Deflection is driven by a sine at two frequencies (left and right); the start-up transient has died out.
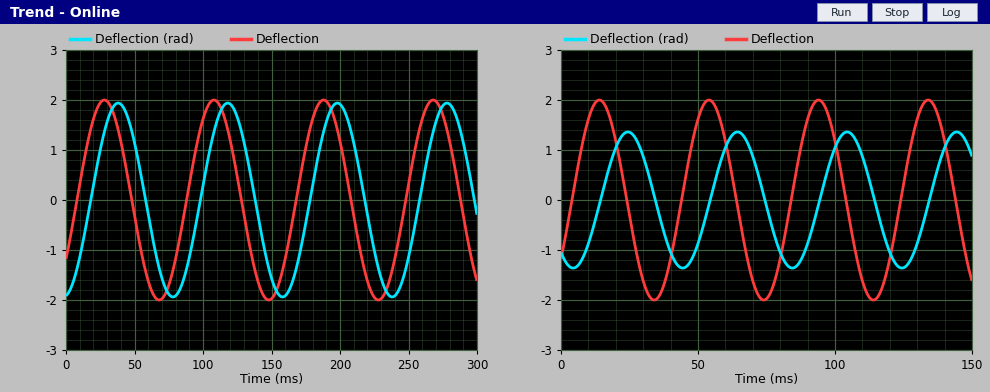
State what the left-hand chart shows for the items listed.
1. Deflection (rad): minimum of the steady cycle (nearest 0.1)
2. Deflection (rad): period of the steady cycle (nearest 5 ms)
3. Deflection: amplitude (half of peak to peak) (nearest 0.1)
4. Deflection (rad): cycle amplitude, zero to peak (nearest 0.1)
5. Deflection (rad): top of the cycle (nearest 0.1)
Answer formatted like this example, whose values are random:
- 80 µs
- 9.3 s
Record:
- -1.9
- 80 ms
- 2.0
- 1.9
- 1.9
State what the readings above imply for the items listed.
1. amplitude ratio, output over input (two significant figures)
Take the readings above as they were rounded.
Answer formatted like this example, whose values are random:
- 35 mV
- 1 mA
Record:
- 0.95
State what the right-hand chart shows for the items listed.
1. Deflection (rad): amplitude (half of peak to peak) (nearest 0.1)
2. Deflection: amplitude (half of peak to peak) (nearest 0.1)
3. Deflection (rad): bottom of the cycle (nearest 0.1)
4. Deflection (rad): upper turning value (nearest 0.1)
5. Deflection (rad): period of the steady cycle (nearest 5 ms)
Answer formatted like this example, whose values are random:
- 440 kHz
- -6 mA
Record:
- 1.4
- 2.0
- -1.4
- 1.4
- 40 ms
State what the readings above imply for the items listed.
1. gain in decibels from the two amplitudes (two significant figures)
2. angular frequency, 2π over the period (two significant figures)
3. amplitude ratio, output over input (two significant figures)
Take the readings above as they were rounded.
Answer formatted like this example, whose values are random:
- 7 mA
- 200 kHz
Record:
- -3.1 dB
- 0.16 rad/ms
- 0.70
